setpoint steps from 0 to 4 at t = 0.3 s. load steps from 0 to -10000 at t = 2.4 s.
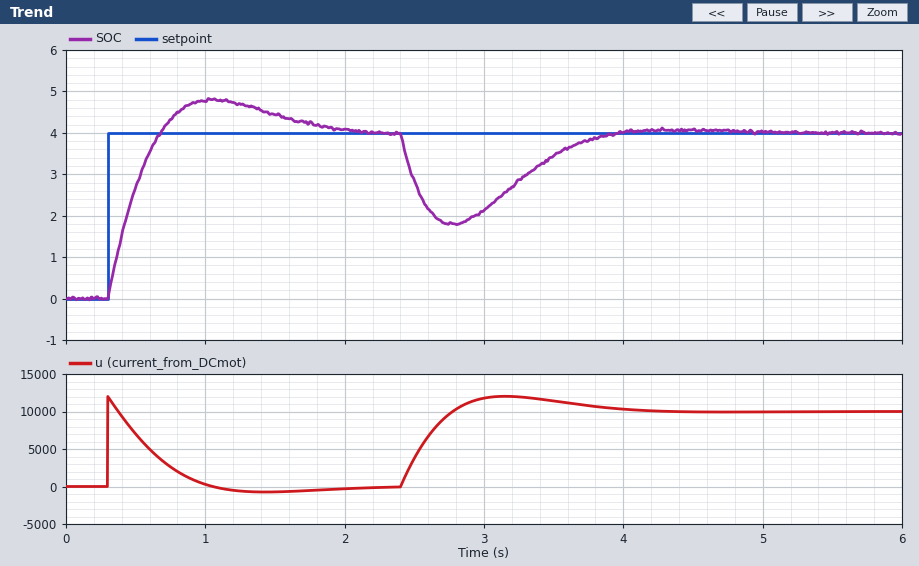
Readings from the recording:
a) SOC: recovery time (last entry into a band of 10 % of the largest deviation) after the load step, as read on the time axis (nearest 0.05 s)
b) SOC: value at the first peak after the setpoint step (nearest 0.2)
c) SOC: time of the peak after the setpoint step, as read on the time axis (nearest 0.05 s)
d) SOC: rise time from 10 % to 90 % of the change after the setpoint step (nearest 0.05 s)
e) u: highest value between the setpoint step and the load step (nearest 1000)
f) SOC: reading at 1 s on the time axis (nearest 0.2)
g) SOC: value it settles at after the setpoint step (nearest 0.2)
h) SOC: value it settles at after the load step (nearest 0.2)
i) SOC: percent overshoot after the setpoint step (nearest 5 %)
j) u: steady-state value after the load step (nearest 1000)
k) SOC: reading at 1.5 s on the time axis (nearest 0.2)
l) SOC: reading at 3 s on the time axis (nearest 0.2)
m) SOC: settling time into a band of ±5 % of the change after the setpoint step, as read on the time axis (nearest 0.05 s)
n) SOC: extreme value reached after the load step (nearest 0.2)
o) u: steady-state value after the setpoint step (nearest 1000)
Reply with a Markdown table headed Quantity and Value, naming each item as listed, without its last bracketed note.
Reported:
| Quantity | Value |
|---|---|
| SOC: recovery time (last entry into a band of 10 % of the largest deviation) after the load step, as read on the time axis | 3.70 s |
| SOC: value at the first peak after the setpoint step | 4.8 |
| SOC: time of the peak after the setpoint step, as read on the time axis | 1.05 s |
| SOC: rise time from 10 % to 90 % of the change after the setpoint step | 0.30 s |
| u: highest value between the setpoint step and the load step | 12000 |
| SOC: reading at 1 s on the time axis | 4.8 |
| SOC: value it settles at after the setpoint step | 4.0 |
| SOC: value it settles at after the load step | 4.0 |
| SOC: percent overshoot after the setpoint step | 20 % |
| u: steady-state value after the load step | 10000 |
| SOC: reading at 1.5 s on the time axis | 4.4 |
| SOC: reading at 3 s on the time axis | 2.2 |
| SOC: settling time into a band of ±5 % of the change after the setpoint step, as read on the time axis | 1.80 s |
| SOC: extreme value reached after the load step | 1.8 |
| u: steady-state value after the setpoint step | 0 |
